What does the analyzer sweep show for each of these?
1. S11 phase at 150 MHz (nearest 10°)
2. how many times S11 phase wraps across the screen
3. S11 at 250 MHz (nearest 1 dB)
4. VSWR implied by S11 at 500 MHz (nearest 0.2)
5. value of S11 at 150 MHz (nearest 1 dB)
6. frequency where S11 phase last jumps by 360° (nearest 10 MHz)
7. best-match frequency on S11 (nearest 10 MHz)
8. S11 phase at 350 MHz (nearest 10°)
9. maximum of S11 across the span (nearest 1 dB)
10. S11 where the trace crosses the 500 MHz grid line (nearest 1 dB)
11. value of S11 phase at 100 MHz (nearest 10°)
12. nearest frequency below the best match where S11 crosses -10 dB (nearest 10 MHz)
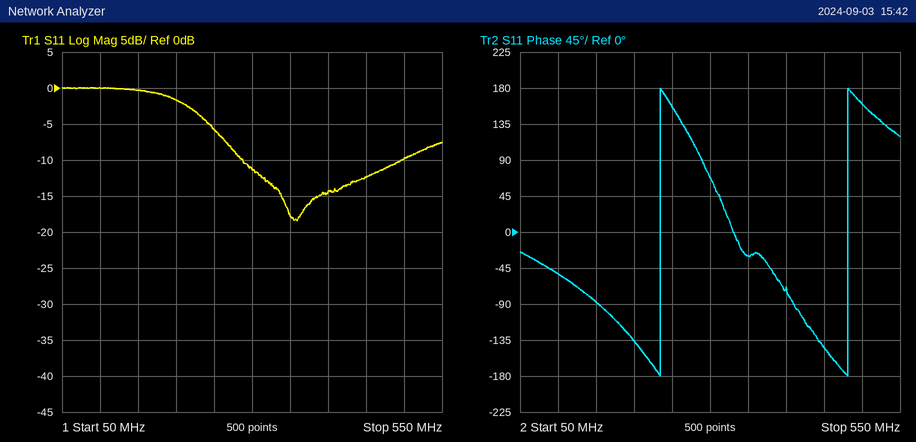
-90°
2
-6 dB
2.0
0 dB
480 MHz
360 MHz
-30°
0 dB
-10 dB
-50°
290 MHz
